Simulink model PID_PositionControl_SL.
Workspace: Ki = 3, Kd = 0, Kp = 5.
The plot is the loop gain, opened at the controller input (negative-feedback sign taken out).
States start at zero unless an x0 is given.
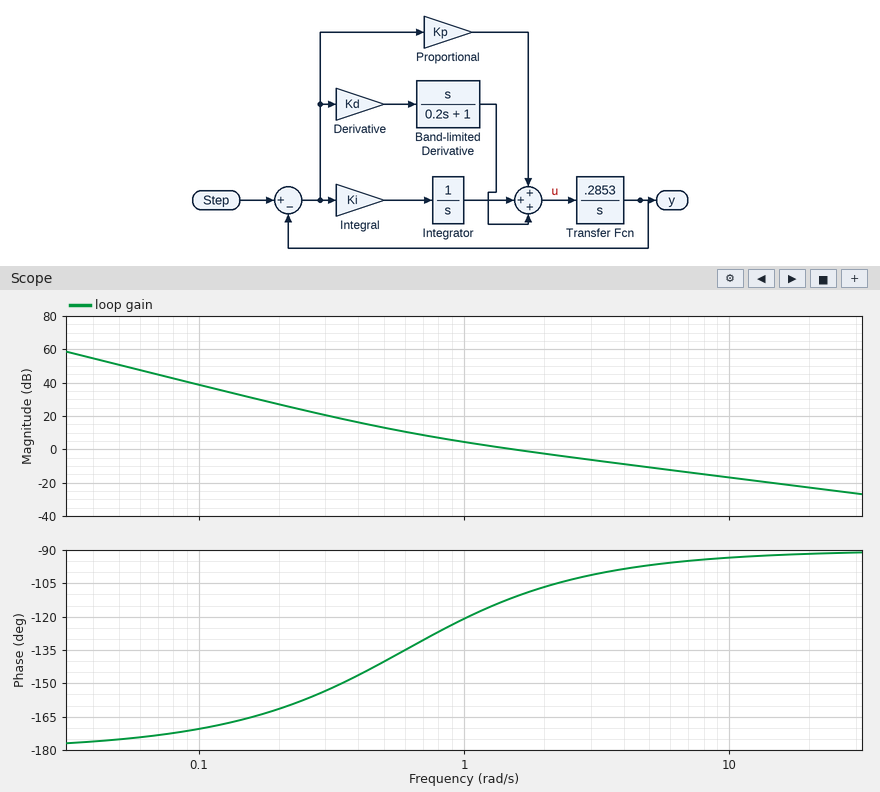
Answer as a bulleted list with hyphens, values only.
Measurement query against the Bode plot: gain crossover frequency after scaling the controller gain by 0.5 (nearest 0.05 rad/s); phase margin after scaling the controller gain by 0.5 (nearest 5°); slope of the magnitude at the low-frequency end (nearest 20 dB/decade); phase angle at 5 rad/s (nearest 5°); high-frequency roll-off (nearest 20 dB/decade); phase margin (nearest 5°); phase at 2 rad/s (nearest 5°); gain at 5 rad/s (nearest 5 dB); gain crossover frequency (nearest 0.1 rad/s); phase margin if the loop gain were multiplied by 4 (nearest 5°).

- 0.85 rad/s
- 55°
- -40 dB/decade
- -95°
- -20 dB/decade
- 70°
- -105°
- -10 dB
- 1.5 rad/s
- 85°
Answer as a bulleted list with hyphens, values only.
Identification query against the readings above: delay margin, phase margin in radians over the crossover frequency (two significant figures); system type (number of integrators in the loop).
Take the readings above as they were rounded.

- 0.81 s
- 2
